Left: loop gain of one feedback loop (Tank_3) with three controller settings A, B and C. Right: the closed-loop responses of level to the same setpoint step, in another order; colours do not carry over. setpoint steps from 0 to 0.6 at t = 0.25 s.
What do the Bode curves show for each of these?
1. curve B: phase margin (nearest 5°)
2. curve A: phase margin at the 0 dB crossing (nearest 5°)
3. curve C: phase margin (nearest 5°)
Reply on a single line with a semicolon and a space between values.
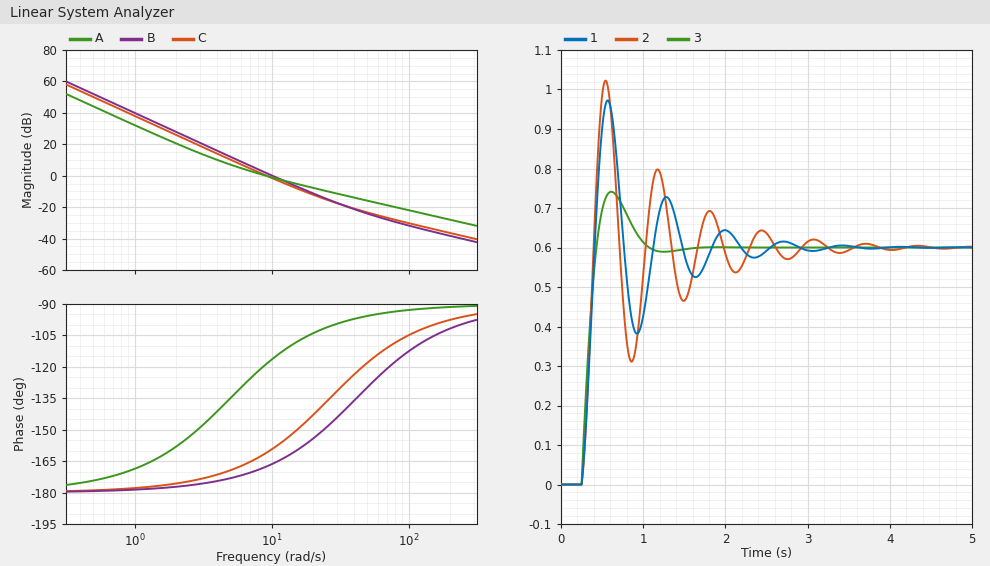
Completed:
15°; 60°; 20°
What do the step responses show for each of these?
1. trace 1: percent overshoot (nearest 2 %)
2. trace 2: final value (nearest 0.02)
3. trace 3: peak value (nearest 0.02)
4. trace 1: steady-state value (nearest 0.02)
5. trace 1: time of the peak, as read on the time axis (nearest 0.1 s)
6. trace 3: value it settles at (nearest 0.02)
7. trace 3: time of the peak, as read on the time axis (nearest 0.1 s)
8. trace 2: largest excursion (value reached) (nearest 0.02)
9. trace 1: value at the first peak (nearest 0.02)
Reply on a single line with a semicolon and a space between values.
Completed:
62 %; 0.60; 0.74; 0.60; 0.6 s; 0.60; 0.6 s; 1.02; 0.98
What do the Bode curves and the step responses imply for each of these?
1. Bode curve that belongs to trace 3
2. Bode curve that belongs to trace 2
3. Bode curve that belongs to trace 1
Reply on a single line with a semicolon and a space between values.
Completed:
A; B; C
